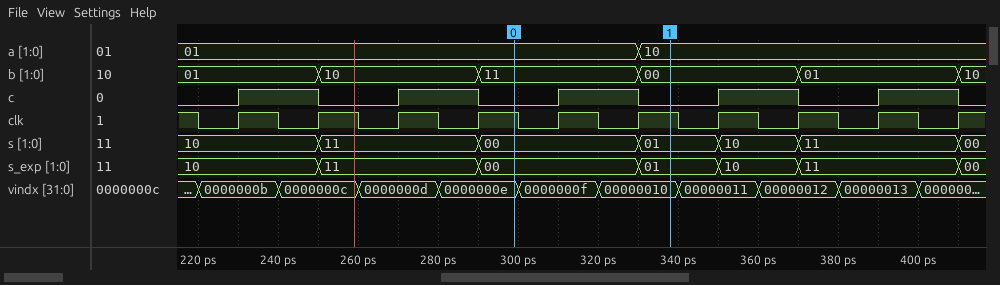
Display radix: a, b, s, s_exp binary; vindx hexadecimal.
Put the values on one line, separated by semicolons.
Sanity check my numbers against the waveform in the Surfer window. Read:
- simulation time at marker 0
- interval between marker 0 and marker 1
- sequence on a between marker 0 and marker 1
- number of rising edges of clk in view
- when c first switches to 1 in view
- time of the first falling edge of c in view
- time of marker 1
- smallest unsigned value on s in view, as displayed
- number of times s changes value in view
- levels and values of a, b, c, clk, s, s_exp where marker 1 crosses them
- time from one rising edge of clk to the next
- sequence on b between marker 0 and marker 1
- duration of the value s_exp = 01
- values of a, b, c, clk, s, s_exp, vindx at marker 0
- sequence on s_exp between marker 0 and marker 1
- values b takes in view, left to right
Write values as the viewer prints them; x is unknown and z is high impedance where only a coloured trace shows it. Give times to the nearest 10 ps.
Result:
300 ps; 40 ps; 01, 10; 10; 230 ps; 250 ps; 340 ps; 00; 6; a=10, b=00, c=0, clk=1, s=01, s_exp=01; 20 ps; 11, 00; 20 ps; a=01, b=11, c=0, clk=1, s=00, s_exp=00, vindx=0000000e; 00, 01; 01, 10, 11, 00, 01, 10
